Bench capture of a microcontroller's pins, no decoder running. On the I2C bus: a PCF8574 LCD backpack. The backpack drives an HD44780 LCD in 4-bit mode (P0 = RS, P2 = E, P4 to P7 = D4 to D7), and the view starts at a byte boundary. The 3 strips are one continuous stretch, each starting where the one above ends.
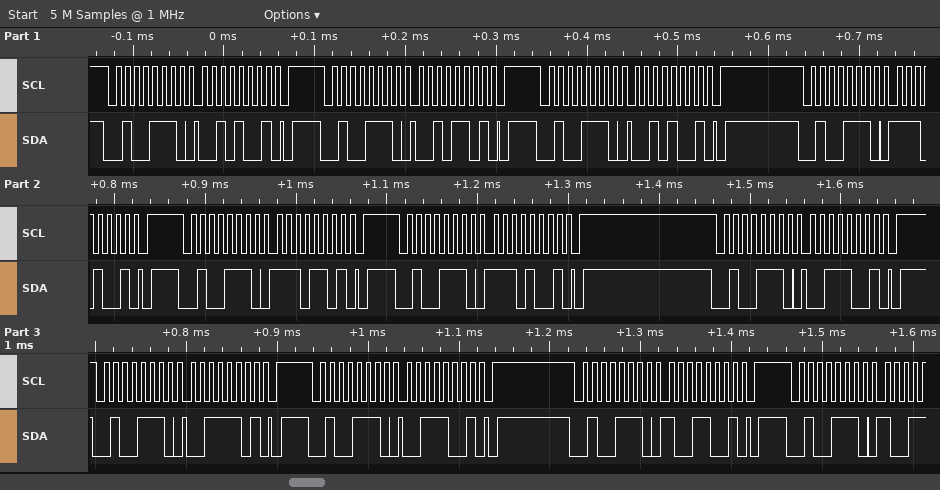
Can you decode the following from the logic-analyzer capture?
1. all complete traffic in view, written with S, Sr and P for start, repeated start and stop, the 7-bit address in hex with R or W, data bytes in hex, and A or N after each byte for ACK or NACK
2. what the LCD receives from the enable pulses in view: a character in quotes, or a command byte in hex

S 27W A 29 A P S 27W A 2D A P S 27W A 29 A P S 27W A E9 A P S 27W A ED A P S 27W A E9 A P S 27W A 39 A P S 27W A 3D A P S 27W A 39 A P S 27W A 99 A P S 27W A
'.'
